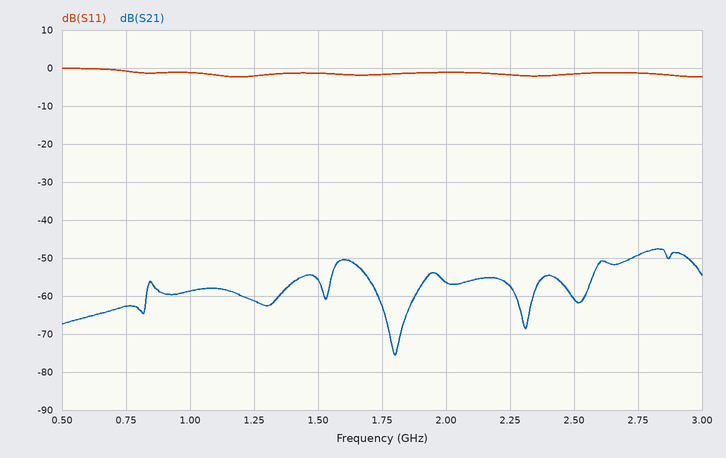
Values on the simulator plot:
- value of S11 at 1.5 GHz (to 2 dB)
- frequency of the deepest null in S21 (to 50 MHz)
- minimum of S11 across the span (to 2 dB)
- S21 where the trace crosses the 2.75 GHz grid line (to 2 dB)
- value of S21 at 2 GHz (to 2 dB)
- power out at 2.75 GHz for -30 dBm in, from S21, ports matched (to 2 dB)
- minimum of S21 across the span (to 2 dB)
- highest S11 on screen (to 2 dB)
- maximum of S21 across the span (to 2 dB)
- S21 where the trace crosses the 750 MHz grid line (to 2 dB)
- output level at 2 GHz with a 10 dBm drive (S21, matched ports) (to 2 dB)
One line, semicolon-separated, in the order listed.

-2 dB; 1.80 GHz; -2 dB; -50 dB; -56 dB; -80 dBm; -76 dB; 0 dB; -48 dB; -62 dB; -46 dBm
